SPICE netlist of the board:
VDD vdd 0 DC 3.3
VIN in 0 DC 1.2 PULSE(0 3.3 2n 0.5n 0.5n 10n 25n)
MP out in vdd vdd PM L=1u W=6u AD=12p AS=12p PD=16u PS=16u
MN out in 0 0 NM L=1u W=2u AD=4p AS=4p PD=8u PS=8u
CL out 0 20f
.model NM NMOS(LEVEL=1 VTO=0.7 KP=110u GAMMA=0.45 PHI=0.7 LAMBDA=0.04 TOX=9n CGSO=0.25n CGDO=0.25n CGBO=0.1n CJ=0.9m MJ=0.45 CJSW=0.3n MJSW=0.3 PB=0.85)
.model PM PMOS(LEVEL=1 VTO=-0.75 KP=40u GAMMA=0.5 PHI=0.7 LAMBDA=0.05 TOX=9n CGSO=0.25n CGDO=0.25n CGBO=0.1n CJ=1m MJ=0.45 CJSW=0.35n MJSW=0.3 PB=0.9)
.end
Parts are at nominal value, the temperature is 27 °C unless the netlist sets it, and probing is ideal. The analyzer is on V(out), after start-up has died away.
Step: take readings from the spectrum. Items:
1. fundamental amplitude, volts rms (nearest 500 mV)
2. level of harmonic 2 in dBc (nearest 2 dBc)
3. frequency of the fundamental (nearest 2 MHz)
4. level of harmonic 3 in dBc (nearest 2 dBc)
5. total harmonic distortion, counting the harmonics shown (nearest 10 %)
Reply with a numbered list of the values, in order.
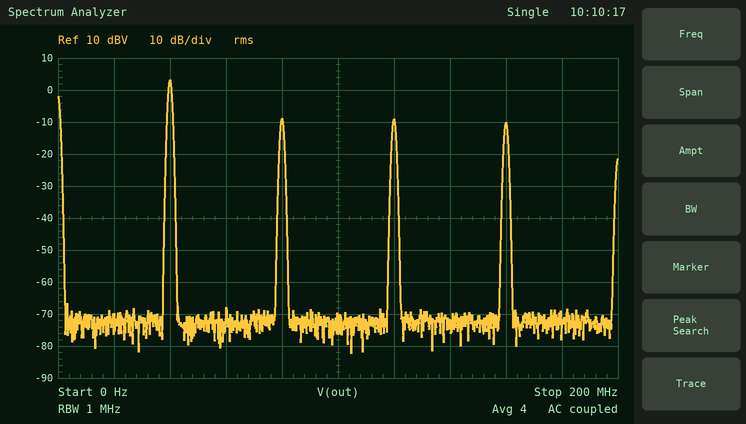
1. 1.5 V
2. -12 dBc
3. 40 MHz
4. -12 dBc
5. 40 %
